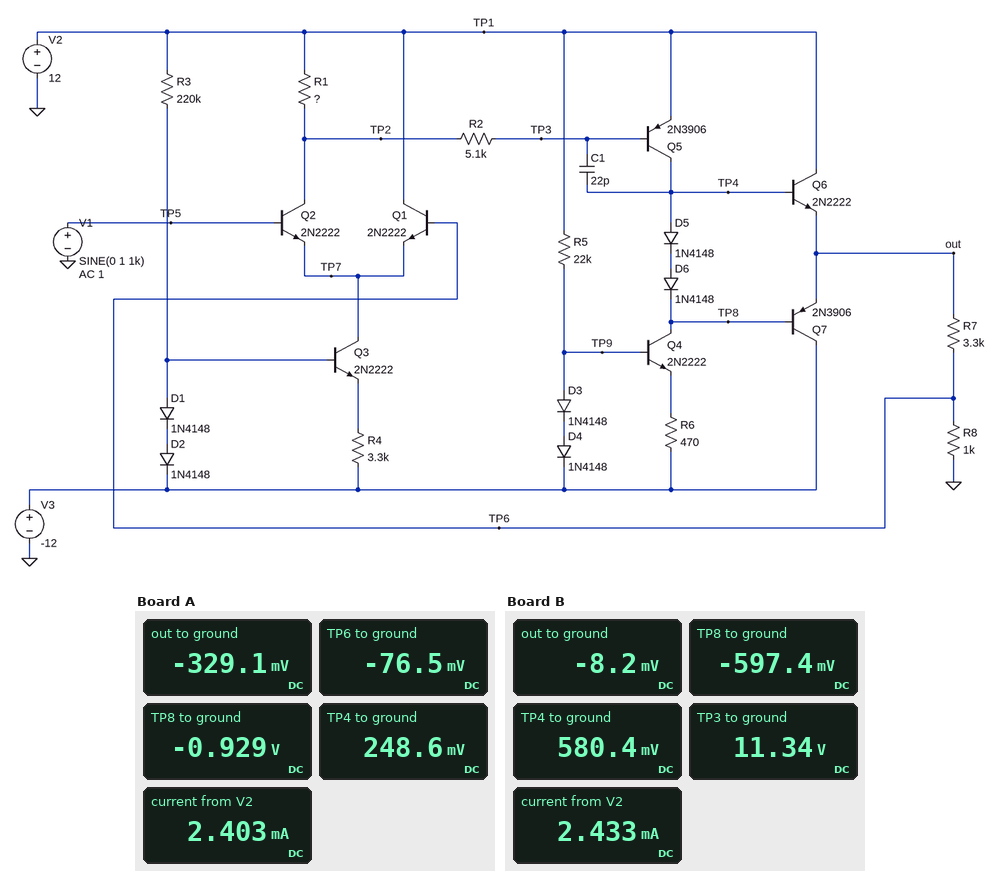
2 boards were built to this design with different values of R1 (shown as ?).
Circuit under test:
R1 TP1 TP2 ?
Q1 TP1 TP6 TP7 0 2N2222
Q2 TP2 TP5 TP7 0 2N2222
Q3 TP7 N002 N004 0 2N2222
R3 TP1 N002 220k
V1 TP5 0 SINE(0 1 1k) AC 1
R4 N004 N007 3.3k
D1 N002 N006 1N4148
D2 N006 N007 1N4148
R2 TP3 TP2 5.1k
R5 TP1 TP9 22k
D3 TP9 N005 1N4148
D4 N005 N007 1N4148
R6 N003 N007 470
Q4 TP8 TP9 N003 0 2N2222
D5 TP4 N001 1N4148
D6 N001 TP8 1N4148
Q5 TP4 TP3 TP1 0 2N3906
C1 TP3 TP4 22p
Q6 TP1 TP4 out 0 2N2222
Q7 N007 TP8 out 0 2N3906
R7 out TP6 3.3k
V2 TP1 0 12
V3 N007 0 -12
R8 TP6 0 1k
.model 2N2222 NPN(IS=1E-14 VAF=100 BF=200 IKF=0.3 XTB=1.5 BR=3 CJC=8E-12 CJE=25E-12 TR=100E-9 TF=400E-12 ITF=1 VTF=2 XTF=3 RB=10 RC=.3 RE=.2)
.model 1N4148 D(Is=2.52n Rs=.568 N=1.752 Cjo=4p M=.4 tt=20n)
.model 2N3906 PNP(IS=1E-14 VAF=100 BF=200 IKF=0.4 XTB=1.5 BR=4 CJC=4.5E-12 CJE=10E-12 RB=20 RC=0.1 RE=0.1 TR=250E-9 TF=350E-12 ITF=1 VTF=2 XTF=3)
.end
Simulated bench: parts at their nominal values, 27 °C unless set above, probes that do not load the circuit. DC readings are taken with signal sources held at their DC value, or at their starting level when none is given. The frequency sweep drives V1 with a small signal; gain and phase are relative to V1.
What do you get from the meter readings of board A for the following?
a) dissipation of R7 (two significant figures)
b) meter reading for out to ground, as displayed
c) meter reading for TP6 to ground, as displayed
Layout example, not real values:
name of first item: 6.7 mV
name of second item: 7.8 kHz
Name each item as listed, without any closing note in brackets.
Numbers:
dissipation of R7: 19 µW
meter reading for out to ground, as displayed: -329.1 mV
meter reading for TP6 to ground, as displayed: -76.5 mV
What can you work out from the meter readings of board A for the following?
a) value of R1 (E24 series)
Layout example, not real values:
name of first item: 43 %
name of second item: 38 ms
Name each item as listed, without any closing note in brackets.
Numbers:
value of R1: 6.8 kΩ
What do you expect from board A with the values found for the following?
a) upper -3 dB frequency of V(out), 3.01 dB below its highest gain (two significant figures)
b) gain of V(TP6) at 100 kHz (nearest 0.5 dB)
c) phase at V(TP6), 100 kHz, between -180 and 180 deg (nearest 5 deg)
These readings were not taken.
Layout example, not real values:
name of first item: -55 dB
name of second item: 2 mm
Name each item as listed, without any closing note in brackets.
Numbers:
upper -3 dB frequency of V(out), 3.01 dB below its highest gain: 160 kHz
gain of V(TP6) at 100 kHz: -1.5 dB
phase at V(TP6), 100 kHz, between -180 and 180 deg: -30 deg
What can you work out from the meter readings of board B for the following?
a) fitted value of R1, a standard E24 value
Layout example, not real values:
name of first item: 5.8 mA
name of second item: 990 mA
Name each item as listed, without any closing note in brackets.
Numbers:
fitted value of R1, a standard E24 value: 13 kΩ
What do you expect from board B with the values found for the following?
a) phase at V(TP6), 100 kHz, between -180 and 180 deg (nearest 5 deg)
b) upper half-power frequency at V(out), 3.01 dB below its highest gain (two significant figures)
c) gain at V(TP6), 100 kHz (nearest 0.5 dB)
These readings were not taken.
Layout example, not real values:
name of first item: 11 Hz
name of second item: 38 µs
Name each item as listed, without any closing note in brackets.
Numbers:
phase at V(TP6), 100 kHz, between -180 and 180 deg: -5 deg
upper half-power frequency at V(out), 3.01 dB below its highest gain: 1.5 MHz
gain at V(TP6), 100 kHz: 0 dB
